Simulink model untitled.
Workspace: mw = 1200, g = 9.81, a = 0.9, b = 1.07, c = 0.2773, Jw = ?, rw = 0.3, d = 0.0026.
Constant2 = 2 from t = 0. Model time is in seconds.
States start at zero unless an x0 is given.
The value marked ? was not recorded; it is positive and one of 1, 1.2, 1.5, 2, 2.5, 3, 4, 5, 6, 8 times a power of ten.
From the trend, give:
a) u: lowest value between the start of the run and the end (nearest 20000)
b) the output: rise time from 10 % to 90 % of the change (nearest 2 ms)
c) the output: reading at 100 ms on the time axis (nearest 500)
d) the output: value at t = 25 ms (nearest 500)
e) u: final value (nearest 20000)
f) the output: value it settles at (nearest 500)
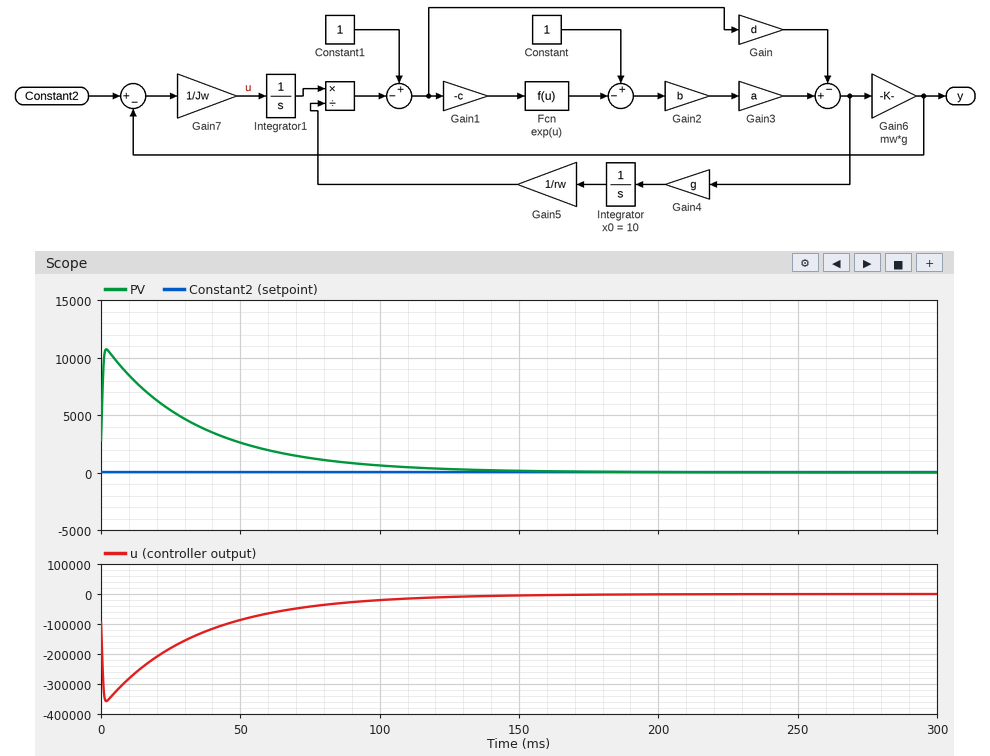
-360000
76 ms
500
5500
0
0
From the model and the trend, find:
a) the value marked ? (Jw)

0.03
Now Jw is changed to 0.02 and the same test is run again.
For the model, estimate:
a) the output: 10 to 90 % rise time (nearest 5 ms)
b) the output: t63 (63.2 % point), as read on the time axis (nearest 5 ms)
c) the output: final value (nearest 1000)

50 ms
55 ms
0
